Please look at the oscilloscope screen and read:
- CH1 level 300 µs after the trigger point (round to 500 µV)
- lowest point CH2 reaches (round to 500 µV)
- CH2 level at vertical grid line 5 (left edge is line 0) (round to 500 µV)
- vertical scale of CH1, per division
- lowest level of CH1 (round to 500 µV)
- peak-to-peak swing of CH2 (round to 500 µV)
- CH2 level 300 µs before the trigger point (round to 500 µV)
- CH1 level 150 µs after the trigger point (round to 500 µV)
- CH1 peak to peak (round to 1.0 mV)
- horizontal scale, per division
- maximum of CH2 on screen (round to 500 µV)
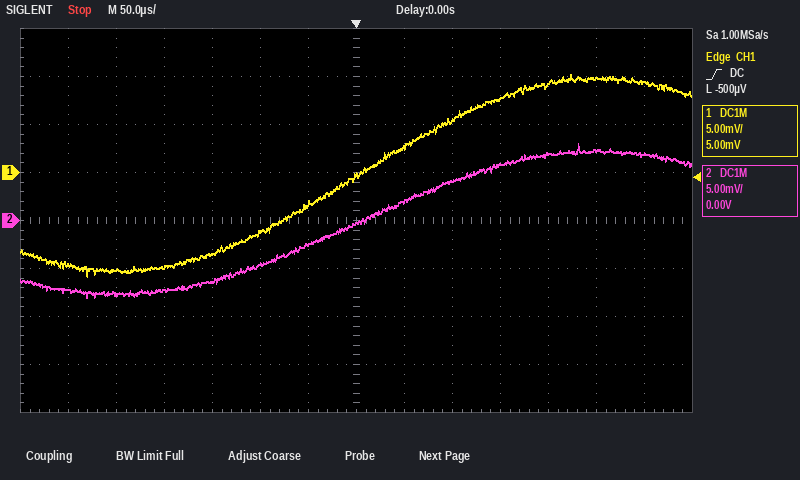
9.5 mV
-8.0 mV
-4.5 mV
5 mV
-11.0 mV
16.0 mV
-7.0 mV
7.5 mV
21.0 mV
50 µs
8.0 mV
